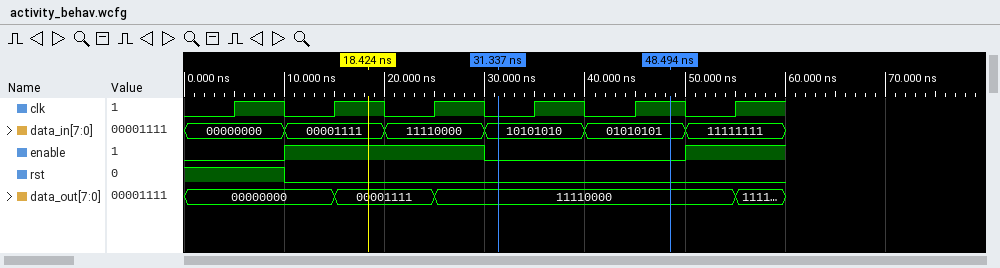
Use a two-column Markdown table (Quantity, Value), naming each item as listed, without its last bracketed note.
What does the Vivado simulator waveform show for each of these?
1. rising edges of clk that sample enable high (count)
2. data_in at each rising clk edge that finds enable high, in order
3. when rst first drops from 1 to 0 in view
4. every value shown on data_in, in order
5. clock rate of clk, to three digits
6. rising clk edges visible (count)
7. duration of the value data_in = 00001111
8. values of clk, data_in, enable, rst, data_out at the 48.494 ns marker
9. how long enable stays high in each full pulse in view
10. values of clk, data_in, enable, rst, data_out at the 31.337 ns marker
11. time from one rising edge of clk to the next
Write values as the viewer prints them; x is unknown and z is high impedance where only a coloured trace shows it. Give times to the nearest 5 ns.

| Quantity | Value |
|---|---|
| rising edges of clk that sample enable high | 3 |
| data_in at each rising clk edge that finds enable high, in order | 00001111, 11110000, 11111111 |
| when rst first drops from 1 to 0 in view | 10 ns |
| every value shown on data_in, in order | 00000000, 00001111, 11110000, 10101010, 01010101, 11111111 |
| clock rate of clk, to three digits | 100 MHz |
| rising clk edges visible | 6 |
| duration of the value data_in = 00001111 | 10 ns |
| values of clk, data_in, enable, rst, data_out at the 48.494 ns marker | clk=1, data_in=01010101, enable=0, rst=0, data_out=11110000 |
| how long enable stays high in each full pulse in view | 20 ns |
| values of clk, data_in, enable, rst, data_out at the 31.337 ns marker | clk=0, data_in=10101010, enable=0, rst=0, data_out=11110000 |
| time from one rising edge of clk to the next | 10 ns |
